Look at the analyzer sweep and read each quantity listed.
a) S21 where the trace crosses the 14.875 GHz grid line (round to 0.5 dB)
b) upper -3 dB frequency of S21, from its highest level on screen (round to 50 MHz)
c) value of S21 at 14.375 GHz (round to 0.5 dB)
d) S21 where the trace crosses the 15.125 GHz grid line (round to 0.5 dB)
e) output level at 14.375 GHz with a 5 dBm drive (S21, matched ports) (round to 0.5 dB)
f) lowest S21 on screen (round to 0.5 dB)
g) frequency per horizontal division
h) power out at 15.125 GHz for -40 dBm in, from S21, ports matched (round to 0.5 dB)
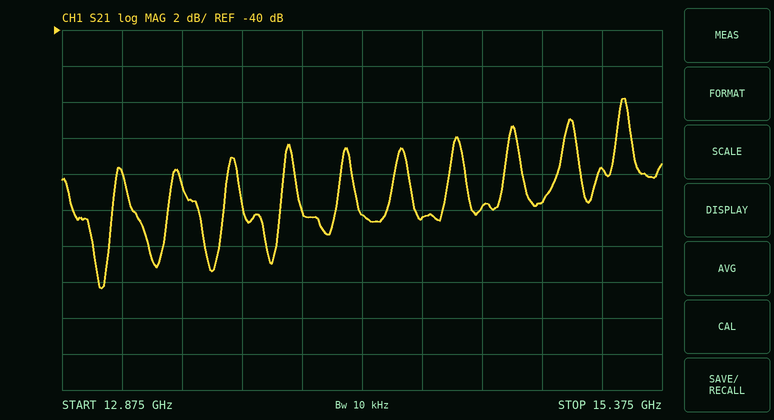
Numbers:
-49.5 dB
15.25 GHz
-50.5 dB
-47.5 dB
-45.5 dBm
-54.5 dB
250 MHz
-87.5 dBm
